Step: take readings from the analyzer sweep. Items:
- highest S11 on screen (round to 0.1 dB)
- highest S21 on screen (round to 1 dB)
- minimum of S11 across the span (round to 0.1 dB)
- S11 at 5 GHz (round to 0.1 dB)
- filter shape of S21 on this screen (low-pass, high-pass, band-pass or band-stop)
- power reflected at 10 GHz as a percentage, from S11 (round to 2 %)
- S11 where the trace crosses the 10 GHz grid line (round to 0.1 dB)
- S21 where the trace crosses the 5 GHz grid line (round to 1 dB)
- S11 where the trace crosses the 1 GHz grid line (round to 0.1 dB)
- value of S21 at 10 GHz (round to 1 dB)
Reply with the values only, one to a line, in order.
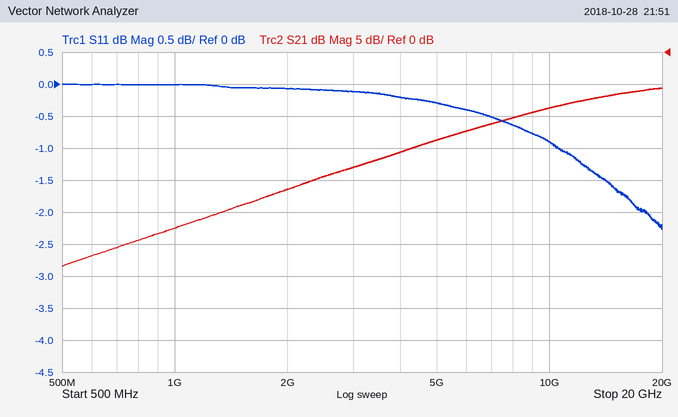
0.0 dB
-6 dB
-2.3 dB
-0.3 dB
high-pass
82 %
-0.9 dB
-14 dB
0.0 dB
-9 dB
